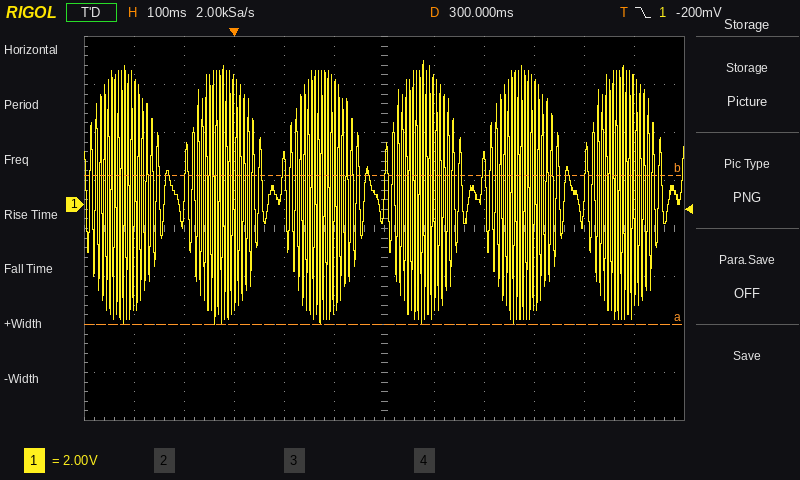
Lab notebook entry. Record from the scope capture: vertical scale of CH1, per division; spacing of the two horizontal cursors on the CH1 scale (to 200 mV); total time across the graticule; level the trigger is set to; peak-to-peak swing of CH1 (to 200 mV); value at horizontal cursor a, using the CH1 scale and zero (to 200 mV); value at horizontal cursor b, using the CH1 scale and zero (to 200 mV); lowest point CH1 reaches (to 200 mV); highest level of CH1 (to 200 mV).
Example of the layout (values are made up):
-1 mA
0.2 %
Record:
2 V
6.2 V
1.2 s
-200 mV
11.0 V
-5.0 V
1.2 V
-5.0 V
6.0 V
